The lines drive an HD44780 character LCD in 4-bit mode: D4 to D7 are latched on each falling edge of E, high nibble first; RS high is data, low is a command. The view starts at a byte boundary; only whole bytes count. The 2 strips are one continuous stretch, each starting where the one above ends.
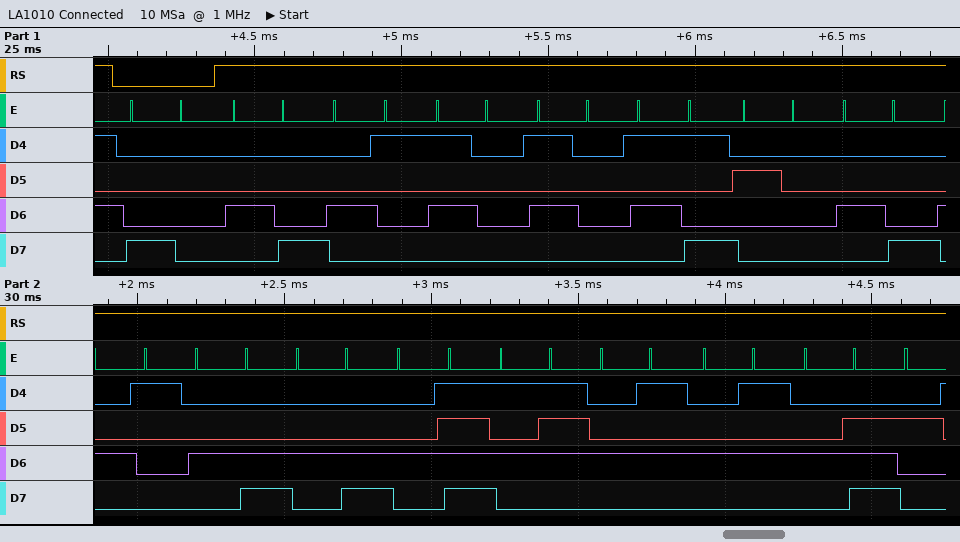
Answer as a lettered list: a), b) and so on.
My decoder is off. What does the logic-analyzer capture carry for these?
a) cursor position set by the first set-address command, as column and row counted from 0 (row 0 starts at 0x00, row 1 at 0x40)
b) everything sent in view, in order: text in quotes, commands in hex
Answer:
a) column 0, row 0
b) 0x80 "HAPPY HALLOWEEN"
